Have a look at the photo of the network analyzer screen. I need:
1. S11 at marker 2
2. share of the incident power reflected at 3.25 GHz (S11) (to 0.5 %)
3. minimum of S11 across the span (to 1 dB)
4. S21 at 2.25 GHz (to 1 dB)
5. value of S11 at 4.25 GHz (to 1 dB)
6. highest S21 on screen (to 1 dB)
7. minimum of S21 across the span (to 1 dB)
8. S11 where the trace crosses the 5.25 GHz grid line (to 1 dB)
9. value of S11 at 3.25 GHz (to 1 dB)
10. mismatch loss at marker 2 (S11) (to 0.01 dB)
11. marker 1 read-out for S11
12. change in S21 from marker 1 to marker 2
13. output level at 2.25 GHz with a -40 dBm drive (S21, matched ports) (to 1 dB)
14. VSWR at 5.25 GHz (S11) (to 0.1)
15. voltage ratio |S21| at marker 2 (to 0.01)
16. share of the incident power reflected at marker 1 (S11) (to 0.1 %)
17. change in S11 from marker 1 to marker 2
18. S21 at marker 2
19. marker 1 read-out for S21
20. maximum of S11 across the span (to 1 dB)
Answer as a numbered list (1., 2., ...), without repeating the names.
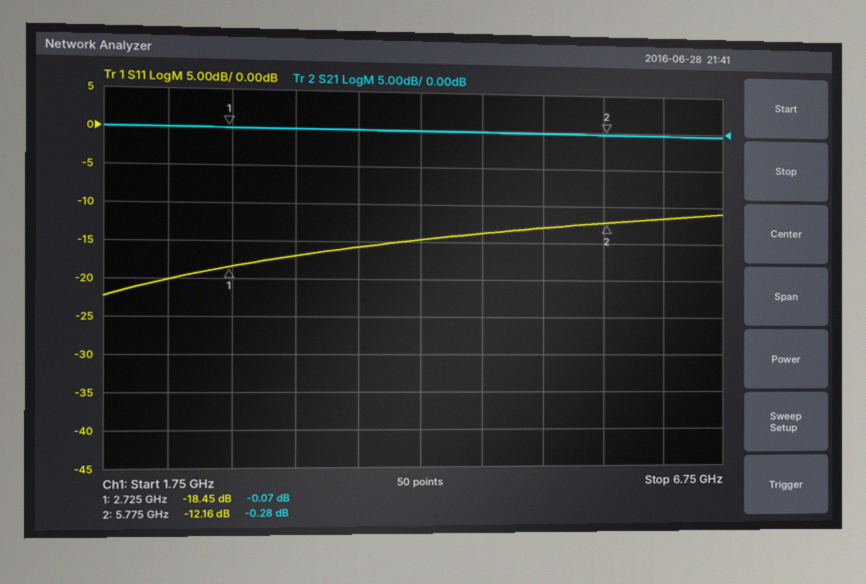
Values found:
1. -12.16 dB
2. 2.0 %
3. -22 dB
4. 0 dB
5. -15 dB
6. 0 dB
7. 0 dB
8. -13 dB
9. -17 dB
10. 0.27 dB
11. -18.45 dB
12. -0.21 dB
13. -40 dBm
14. 1.6
15. 0.97
16. 1.4 %
17. 6.29 dB
18. -0.28 dB
19. -0.07 dB
20. -11 dB
